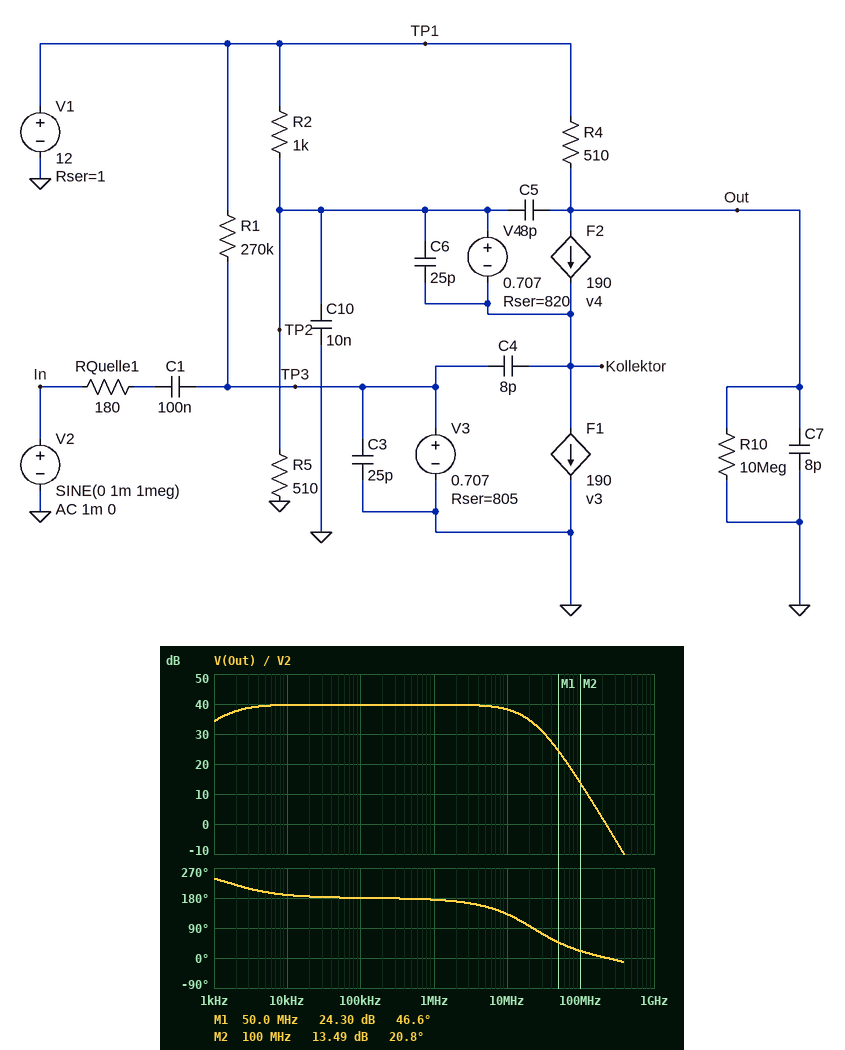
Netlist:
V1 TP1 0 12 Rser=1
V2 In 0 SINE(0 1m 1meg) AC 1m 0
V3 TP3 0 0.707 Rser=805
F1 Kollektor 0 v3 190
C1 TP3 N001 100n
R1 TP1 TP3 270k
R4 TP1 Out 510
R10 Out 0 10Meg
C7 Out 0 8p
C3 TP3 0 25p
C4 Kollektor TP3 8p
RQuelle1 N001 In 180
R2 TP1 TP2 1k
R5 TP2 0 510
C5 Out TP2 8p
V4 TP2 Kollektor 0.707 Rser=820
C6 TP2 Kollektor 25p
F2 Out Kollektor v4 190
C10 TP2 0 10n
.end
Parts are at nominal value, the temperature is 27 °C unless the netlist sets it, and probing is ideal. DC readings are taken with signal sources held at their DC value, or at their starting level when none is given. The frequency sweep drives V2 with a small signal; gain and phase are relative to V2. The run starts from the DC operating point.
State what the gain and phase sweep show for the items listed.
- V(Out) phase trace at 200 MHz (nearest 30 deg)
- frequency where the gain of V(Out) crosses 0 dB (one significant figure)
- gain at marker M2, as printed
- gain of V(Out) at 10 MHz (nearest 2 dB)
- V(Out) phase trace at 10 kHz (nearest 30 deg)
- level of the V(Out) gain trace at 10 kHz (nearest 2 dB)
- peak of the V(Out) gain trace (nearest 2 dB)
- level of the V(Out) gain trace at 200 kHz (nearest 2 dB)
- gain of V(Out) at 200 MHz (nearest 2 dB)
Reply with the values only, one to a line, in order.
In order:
0 deg
200 MHz
13.49 dB
38 dB
180 deg
40 dB
40 dB
40 dB
2 dB
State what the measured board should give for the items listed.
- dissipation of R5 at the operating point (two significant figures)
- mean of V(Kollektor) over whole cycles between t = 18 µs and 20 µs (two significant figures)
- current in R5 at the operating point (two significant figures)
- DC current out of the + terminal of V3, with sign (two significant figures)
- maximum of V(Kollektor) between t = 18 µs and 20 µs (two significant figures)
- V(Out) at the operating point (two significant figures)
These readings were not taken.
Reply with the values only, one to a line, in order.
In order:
32 mW
3.3 V
7.9 mA
-42 µA
3.3 V
8.0 V
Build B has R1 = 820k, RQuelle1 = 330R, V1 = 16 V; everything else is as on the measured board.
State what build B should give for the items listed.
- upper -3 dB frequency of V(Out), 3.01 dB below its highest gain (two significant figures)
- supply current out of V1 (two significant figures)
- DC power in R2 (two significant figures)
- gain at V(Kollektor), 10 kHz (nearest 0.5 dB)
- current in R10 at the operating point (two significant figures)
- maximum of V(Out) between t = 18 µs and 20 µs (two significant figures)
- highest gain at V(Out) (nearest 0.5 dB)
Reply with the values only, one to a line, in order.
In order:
11 MHz
14 mA
110 mW
0.5 dB
1.4 µA
14 V
38.5 dB
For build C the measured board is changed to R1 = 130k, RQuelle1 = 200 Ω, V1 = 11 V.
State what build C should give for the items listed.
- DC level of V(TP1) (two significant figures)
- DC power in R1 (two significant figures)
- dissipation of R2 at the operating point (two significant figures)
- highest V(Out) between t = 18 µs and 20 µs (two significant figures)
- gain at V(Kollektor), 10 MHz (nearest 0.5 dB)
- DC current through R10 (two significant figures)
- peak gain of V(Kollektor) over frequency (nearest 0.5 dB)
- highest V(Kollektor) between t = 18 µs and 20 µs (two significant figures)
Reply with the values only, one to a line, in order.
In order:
11 V
800 µW
53 mW
3.5 V
-2.0 dB
340 nA
1.5 dB
2.9 V
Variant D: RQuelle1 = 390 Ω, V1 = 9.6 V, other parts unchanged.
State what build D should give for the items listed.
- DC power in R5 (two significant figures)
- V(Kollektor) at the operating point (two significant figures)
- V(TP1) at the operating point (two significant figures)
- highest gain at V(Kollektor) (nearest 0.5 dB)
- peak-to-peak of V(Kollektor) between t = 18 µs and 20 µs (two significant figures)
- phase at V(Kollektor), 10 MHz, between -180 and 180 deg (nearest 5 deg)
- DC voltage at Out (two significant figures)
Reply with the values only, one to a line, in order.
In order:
20 mW
2.5 V
9.6 V
0 dB
1.5 mV
145 deg
6.4 V
